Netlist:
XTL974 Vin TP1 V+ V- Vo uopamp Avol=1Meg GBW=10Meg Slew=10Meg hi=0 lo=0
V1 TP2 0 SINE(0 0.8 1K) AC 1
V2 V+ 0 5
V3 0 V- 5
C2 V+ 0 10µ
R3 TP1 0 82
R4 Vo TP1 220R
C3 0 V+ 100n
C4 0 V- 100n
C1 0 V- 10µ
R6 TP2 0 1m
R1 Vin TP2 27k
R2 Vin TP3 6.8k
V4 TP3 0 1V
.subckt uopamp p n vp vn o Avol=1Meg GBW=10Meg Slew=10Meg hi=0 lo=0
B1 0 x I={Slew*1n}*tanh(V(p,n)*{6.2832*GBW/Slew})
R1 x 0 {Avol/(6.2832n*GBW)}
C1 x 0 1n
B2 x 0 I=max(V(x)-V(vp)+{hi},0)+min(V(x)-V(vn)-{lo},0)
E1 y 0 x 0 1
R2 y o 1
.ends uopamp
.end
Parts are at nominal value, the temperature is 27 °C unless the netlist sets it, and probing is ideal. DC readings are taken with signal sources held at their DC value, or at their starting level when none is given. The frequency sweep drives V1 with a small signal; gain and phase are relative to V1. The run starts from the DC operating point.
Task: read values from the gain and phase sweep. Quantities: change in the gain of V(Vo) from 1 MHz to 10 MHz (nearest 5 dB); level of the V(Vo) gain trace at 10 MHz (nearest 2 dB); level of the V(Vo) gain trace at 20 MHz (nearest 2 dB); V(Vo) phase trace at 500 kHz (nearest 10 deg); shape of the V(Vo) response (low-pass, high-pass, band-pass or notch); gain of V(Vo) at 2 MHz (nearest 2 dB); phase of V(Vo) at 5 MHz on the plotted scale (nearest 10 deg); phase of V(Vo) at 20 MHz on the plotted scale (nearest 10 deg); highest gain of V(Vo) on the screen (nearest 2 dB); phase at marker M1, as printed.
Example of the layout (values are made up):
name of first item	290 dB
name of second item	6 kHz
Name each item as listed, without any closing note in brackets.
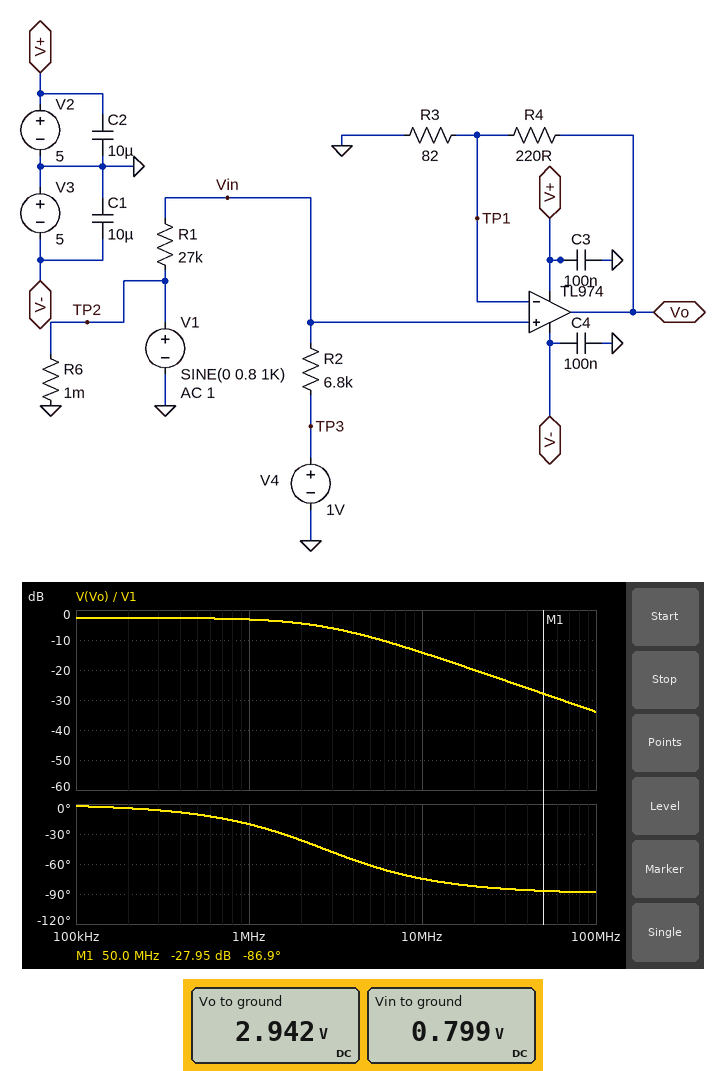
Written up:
change in the gain of V(Vo) from 1 MHz to 10 MHz	-10 dB
level of the V(Vo) gain trace at 10 MHz	-14 dB
level of the V(Vo) gain trace at 20 MHz	-20 dB
V(Vo) phase trace at 500 kHz	-10 deg
shape of the V(Vo) response	low-pass
gain of V(Vo) at 2 MHz	-4 dB
phase of V(Vo) at 5 MHz on the plotted scale	-60 deg
phase of V(Vo) at 20 MHz on the plotted scale	-80 deg
highest gain of V(Vo) on the screen	-2 dB
phase at marker M1, as printed	-86.9 deg
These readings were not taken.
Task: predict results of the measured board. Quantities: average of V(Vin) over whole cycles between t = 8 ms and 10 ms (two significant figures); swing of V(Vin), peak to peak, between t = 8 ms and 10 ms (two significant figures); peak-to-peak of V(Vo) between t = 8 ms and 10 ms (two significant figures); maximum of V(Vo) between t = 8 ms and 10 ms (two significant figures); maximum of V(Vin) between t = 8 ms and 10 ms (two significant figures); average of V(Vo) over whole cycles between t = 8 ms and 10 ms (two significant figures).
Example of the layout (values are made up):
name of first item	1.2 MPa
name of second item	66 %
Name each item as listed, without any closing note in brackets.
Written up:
average of V(Vin) over whole cycles between t = 8 ms and 10 ms	800 mV
swing of V(Vin), peak to peak, between t = 8 ms and 10 ms	320 mV
peak-to-peak of V(Vo) between t = 8 ms and 10 ms	1.2 V
maximum of V(Vo) between t = 8 ms and 10 ms	3.5 V
maximum of V(Vin) between t = 8 ms and 10 ms	960 mV
average of V(Vo) over whole cycles between t = 8 ms and 10 ms	2.9 V
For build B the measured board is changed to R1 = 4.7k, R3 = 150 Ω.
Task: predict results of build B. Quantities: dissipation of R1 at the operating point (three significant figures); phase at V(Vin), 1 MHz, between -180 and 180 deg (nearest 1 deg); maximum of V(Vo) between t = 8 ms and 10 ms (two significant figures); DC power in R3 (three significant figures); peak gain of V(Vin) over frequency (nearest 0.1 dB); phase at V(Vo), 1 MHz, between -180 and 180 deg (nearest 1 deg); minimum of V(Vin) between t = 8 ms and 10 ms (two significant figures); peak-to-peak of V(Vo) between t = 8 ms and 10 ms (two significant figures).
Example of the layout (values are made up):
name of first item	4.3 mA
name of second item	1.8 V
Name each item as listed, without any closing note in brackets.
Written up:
dissipation of R1 at the operating point	35.5 µW
phase at V(Vin), 1 MHz, between -180 and 180 deg	0 deg
maximum of V(Vo) between t = 8 ms and 10 ms	2.2 V
DC power in R3	1.11 mW
peak gain of V(Vin) over frequency	-4.6 dB
phase at V(Vo), 1 MHz, between -180 and 180 deg	-14 deg
minimum of V(Vin) between t = 8 ms and 10 ms	-64 mV
peak-to-peak of V(Vo) between t = 8 ms and 10 ms	2.3 V
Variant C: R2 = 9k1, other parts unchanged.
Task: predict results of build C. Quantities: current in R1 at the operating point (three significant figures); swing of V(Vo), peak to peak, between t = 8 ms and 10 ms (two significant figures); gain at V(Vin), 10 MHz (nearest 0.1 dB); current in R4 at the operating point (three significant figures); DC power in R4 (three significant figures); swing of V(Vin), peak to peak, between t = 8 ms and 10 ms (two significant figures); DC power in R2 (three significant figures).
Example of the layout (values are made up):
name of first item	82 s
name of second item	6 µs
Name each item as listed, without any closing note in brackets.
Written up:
current in R1 at the operating point	27.7 µA
swing of V(Vo), peak to peak, between t = 8 ms and 10 ms	1.5 V
gain at V(Vin), 10 MHz	-12.0 dB
current in R4 at the operating point	9.12 mA
DC power in R4	18.3 mW
swing of V(Vin), peak to peak, between t = 8 ms and 10 ms	400 mV
DC power in R2	6.98 µW
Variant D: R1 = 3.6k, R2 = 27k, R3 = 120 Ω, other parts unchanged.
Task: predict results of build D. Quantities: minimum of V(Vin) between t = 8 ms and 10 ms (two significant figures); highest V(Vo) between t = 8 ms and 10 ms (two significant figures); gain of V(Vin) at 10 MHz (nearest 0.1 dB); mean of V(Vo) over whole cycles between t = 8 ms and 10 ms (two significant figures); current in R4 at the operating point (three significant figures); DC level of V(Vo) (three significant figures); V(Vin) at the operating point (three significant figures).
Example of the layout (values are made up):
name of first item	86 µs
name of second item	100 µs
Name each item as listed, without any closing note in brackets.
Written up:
minimum of V(Vin) between t = 8 ms and 10 ms	-590 mV
highest V(Vo) between t = 8 ms and 10 ms	2.3 V
gain of V(Vin) at 10 MHz	-1.1 dB
mean of V(Vo) over whole cycles between t = 8 ms and 10 ms	330 mV
current in R4 at the operating point	980 µA
DC level of V(Vo)	333 mV
V(Vin) at the operating point	118 mV
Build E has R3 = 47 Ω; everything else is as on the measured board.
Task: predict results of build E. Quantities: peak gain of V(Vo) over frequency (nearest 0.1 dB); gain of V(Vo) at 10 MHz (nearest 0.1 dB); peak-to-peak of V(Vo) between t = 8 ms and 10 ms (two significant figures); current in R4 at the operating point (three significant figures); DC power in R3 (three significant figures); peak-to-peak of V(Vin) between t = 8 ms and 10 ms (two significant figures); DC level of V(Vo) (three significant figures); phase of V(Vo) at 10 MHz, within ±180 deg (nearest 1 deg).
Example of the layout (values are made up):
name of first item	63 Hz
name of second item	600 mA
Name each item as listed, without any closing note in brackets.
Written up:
peak gain of V(Vo) over frequency	1.2 dB
gain of V(Vo) at 10 MHz	-14.1 dB
peak-to-peak of V(Vo) between t = 8 ms and 10 ms	1.4 V
current in R4 at the operating point	17.0 mA
DC power in R3	13.6 mW
peak-to-peak of V(Vin) between t = 8 ms and 10 ms	320 mV
DC level of V(Vo)	4.54 V
phase of V(Vo) at 10 MHz, within ±180 deg	-80 deg
